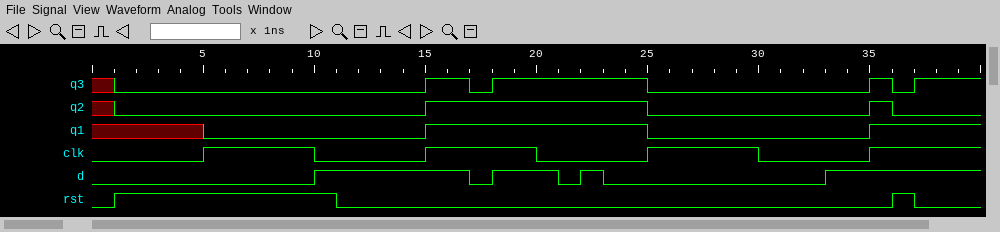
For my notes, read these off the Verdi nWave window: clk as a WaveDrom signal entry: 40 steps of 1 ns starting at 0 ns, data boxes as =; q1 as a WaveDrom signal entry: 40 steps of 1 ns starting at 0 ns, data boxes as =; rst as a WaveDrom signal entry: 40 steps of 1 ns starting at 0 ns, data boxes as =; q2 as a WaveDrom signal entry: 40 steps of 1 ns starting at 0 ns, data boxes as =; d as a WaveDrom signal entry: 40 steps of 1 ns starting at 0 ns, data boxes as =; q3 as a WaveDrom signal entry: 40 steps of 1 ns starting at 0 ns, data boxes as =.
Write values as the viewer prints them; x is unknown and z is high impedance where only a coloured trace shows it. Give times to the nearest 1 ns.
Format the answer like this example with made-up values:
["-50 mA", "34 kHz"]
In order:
["{name: 'clk', wave: '0....1....0....1....0....1....0....1....'}", "{name: 'q1', wave: 'x....0.........1.........0.........1....'}", "{name: 'rst', wave: '01.........0........................10..'}", "{name: 'q2', wave: 'x0.............1.........0.........10...'}", "{name: 'd', wave: '0.........1......01..010.........1......'}", "{name: 'q3', wave: 'x0.............1.01......0.........101..'}"]
